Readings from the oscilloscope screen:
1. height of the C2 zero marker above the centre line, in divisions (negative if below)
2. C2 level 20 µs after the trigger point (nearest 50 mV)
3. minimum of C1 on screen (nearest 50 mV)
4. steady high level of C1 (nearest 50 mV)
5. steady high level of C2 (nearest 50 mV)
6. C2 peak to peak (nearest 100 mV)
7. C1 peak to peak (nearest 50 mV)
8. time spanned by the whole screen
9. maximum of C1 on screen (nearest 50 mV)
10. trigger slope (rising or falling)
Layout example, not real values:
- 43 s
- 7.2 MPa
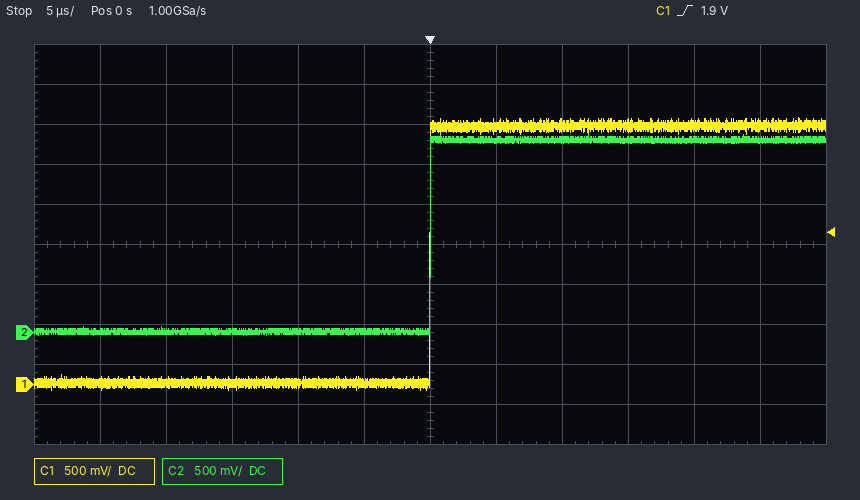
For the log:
- -2.2 div
- 2.40 V
- -50 mV
- 3.25 V
- 2.40 V
- 2.50 V
- 3.40 V
- 60 µs
- 3.35 V
- rising
